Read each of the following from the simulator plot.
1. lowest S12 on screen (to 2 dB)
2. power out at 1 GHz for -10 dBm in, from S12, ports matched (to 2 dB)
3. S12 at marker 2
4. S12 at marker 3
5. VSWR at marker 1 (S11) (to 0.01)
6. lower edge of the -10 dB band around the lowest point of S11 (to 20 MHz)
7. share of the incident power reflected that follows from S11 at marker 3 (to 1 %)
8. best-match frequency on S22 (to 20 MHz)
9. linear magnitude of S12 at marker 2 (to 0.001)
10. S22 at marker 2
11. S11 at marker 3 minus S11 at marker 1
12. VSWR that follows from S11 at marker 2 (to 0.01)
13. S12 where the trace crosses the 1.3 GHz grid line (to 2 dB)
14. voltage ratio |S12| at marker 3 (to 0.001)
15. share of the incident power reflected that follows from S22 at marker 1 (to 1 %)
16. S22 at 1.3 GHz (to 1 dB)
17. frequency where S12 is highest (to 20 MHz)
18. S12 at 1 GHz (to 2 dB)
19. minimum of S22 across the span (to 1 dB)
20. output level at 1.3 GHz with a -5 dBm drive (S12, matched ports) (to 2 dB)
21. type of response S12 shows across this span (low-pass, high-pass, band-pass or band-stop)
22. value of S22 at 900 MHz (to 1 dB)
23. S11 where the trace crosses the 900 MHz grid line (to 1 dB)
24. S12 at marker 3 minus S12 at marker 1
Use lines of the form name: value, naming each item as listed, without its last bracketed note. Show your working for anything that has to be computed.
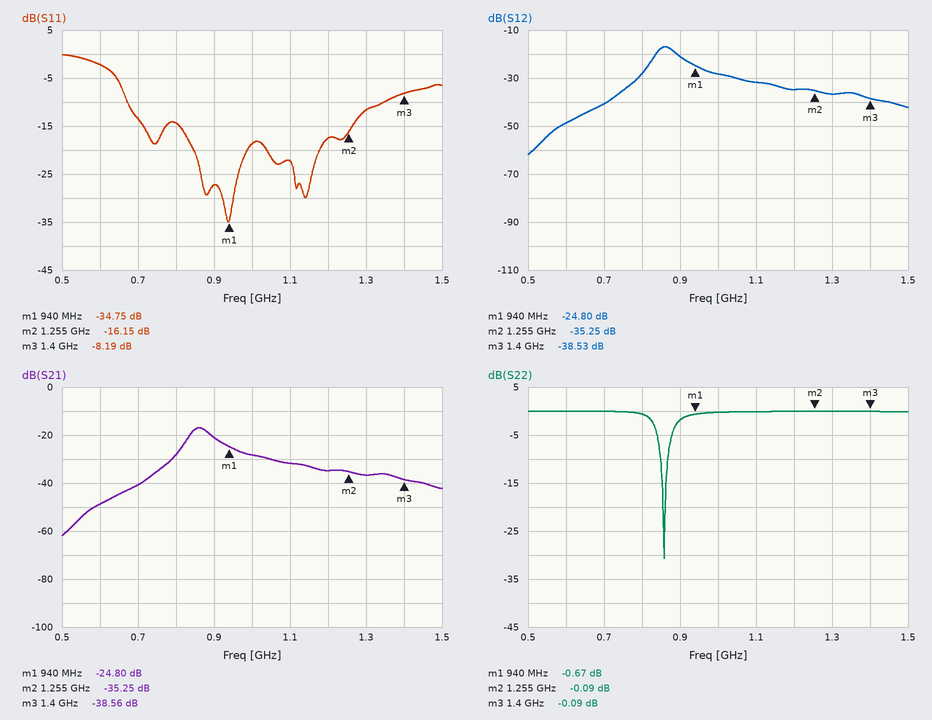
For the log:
lowest S12 on screen: -62 dB
power out at 1 GHz for -10 dBm in, from S12, ports matched: -10 dBm + (-28 dB) = -38 dBm
S12 at marker 2: -35.25 dB
S12 at marker 3: -38.53 dB
VSWR at marker 1 (S11): (1 + 0.0183)/(1 − 0.0183) ≈ 1.04
lower edge of the -10 dB band around the lowest point of S11: 680 MHz
share of the incident power reflected that follows from S11 at marker 3: 10^(-8.19/10) ≈ 15 %
best-match frequency on S22: 860 MHz
linear magnitude of S12 at marker 2: 10^(-35.25/20) ≈ 0.017
S22 at marker 2: -0.09 dB
S11 at marker 3 minus S11 at marker 1: -8.19 − (-34.75) = 26.56 dB
VSWR that follows from S11 at marker 2: (1 + 0.1558)/(1 − 0.1558) ≈ 1.37
S12 where the trace crosses the 1.3 GHz grid line: -36 dB
voltage ratio |S12| at marker 3: 10^(-38.53/20) ≈ 0.012
share of the incident power reflected that follows from S22 at marker 1: 10^(-0.67/10) ≈ 86 %
S22 at 1.3 GHz: 0 dB
frequency where S12 is highest: 860 MHz
S12 at 1 GHz: -28 dB
minimum of S22 across the span: -31 dB
output level at 1.3 GHz with a -5 dBm drive (S12, matched ports): -5 dBm + (-36 dB) = -42 dBm
type of response S12 shows across this span: band-pass
value of S22 at 900 MHz: -2 dB
S11 where the trace crosses the 900 MHz grid line: -27 dB
S12 at marker 3 minus S12 at marker 1: -38.53 − (-24.8) = -13.73 dB
